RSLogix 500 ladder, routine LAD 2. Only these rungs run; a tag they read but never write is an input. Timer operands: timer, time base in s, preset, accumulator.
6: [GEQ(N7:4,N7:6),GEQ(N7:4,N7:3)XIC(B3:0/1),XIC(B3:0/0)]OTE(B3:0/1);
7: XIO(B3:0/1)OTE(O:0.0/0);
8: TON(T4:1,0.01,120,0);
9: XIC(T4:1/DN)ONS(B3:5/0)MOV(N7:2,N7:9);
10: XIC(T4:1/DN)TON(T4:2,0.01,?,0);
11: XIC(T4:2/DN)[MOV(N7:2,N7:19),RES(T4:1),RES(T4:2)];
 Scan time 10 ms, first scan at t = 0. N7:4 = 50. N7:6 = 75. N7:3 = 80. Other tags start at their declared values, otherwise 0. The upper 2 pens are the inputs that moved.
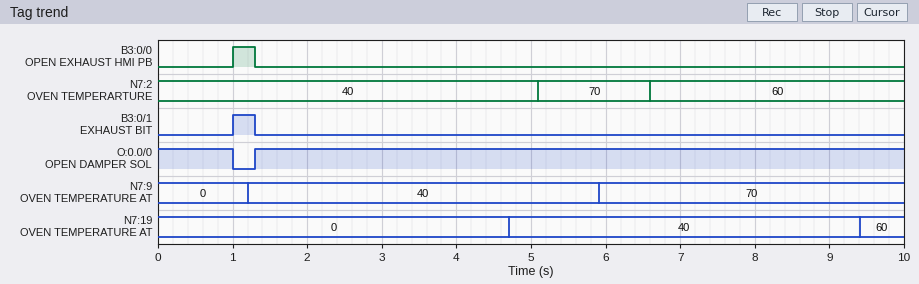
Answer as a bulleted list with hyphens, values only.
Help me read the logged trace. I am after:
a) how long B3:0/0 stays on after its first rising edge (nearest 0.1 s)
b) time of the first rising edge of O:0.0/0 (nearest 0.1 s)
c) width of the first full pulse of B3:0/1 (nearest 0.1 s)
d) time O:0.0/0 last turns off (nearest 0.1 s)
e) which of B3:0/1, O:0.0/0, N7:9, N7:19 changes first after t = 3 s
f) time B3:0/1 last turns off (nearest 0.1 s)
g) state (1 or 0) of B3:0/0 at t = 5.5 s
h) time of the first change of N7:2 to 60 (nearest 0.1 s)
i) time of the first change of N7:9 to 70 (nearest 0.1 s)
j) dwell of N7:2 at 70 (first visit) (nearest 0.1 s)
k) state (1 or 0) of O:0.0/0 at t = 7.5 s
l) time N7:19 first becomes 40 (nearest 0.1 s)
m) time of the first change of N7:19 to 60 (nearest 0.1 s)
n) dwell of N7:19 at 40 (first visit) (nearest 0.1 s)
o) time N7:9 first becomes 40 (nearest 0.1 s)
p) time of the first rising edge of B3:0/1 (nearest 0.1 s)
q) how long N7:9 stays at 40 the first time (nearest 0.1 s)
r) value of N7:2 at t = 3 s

- 0.3 s
- 1.3 s
- 0.3 s
- 1.0 s
- N7:19
- 1.3 s
- 0
- 6.6 s
- 5.9 s
- 1.5 s
- 1
- 4.7 s
- 9.4 s
- 4.7 s
- 1.2 s
- 1.0 s
- 4.7 s
- 40
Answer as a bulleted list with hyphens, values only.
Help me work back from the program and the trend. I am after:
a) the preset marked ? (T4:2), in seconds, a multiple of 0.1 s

- 3.5 s
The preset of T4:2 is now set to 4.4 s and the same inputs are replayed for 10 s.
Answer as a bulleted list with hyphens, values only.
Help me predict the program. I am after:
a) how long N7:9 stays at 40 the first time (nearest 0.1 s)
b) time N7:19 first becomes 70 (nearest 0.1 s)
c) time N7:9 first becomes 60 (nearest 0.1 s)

- 5.6 s
- 5.6 s
- 6.8 s
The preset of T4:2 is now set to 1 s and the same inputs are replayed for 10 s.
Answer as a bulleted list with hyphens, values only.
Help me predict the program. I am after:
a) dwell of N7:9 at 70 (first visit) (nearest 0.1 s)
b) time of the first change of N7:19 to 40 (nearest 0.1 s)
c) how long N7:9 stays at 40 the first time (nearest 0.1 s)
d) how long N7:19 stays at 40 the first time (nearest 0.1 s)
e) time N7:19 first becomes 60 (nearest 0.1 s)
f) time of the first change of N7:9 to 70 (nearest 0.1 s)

- 2.2 s
- 2.2 s
- 4.4 s
- 4.4 s
- 6.6 s
- 5.6 s
